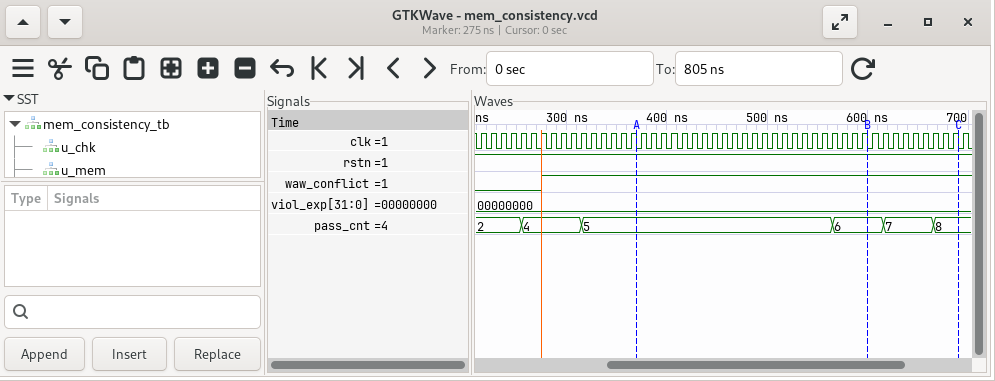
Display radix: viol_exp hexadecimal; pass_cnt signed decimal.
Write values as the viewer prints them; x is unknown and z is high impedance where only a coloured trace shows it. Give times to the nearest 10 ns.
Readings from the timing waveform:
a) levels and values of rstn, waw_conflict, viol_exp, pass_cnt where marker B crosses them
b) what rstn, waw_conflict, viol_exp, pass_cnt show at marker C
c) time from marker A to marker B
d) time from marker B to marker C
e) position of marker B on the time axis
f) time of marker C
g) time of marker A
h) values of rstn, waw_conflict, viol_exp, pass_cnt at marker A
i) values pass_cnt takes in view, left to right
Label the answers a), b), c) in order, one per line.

a) rstn=1, waw_conflict=1, viol_exp=00000000, pass_cnt=6
b) rstn=1, waw_conflict=1, viol_exp=00000000, pass_cnt=8
c) 230 ns
d) 90 ns
e) 600 ns
f) 690 ns
g) 370 ns
h) rstn=1, waw_conflict=1, viol_exp=00000000, pass_cnt=5
i) 2, 4, 5, 6, 7, 8
